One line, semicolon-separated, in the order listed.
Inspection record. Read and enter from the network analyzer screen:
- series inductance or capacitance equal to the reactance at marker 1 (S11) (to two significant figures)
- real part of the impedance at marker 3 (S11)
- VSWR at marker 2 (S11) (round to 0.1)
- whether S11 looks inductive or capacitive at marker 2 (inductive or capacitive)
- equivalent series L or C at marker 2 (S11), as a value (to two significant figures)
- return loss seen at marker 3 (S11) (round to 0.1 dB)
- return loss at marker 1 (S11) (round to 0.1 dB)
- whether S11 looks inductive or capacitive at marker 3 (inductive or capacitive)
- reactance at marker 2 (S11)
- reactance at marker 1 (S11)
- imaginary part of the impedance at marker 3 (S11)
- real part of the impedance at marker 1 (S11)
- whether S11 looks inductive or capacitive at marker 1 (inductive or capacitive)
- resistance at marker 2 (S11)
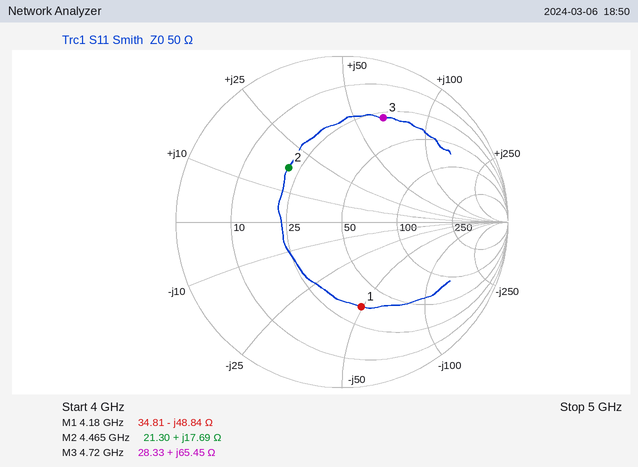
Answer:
780 fF; 28.33 Ω; 2.7; inductive; 630 pH; 3.4 dB; 5.6 dB; inductive; +17.69 Ω; -48.84 Ω; +65.45 Ω; 34.81 Ω; capacitive; 21.30 Ω
